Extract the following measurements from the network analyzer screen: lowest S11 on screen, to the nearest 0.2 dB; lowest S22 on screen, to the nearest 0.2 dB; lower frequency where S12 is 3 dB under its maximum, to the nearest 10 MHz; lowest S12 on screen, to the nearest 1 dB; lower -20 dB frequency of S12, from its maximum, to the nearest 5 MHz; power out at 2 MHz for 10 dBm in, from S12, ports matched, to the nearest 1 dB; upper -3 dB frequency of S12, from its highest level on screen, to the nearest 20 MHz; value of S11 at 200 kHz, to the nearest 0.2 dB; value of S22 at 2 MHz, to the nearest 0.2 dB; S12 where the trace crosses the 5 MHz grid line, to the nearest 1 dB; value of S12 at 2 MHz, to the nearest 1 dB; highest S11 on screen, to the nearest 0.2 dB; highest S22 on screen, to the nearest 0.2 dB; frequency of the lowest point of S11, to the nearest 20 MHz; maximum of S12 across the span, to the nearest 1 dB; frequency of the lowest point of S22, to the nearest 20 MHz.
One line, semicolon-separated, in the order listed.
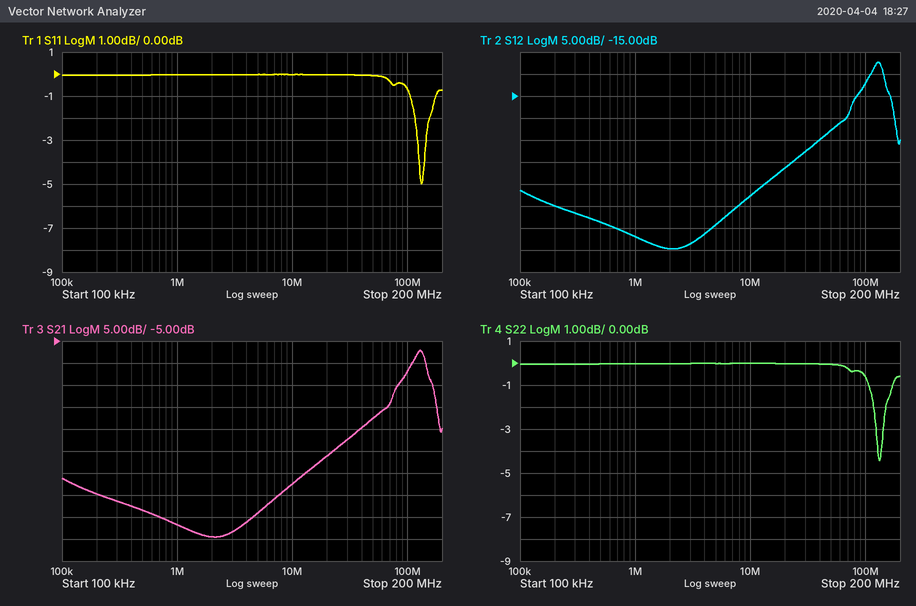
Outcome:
-5.0 dB; -4.4 dB; 110 MHz; -50 dB; 30 MHz; -40 dBm; 140 MHz; 0.0 dB; 0.0 dB; -44 dB; -50 dB; 0.0 dB; 0.0 dB; 140 MHz; -7 dB; 140 MHz
